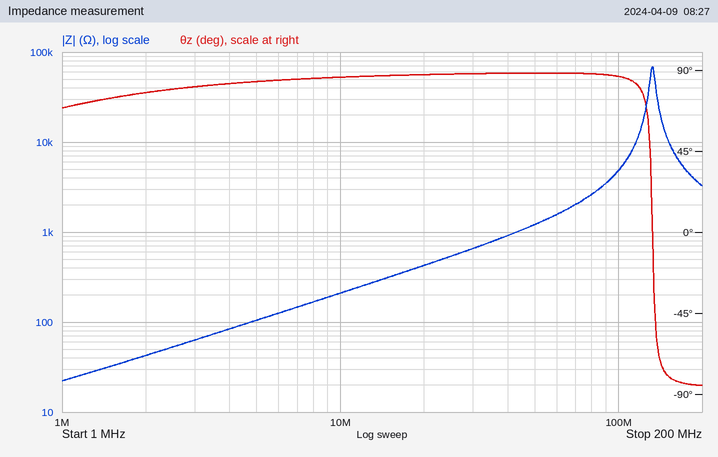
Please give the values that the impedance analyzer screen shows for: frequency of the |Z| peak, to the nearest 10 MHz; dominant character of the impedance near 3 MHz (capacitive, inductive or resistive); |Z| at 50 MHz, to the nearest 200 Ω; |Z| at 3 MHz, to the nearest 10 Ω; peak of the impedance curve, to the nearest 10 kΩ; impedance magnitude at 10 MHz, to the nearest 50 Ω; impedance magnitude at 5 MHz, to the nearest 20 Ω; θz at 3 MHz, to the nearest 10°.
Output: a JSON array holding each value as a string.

["130 MHz", "inductive", "1.2 kΩ", "60 Ω", "70 kΩ", "200 Ω", "100 Ω", "80°"]
